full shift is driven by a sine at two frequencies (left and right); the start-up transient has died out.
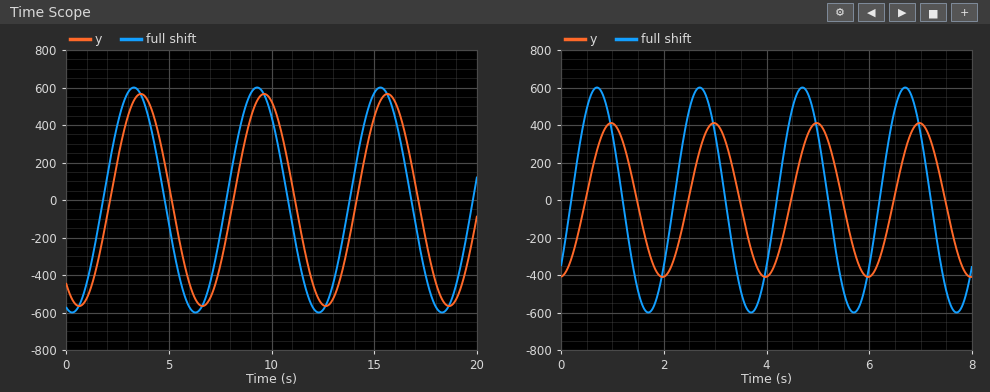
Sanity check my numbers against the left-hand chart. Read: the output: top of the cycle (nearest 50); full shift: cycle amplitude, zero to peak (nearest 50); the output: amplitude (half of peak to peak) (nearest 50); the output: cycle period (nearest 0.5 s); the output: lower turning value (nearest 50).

550
600
550
6.0 s
-550
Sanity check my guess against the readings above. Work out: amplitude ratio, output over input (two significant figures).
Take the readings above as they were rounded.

0.92
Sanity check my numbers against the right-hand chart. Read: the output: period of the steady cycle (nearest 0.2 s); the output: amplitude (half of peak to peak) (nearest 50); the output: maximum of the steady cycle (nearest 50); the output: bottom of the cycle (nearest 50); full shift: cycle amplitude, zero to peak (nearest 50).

2.0 s
400
400
-400
600
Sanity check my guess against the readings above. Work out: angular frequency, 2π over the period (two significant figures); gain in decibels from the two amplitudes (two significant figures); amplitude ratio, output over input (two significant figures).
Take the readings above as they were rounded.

3.1 rad/s
-3.5 dB
0.67
